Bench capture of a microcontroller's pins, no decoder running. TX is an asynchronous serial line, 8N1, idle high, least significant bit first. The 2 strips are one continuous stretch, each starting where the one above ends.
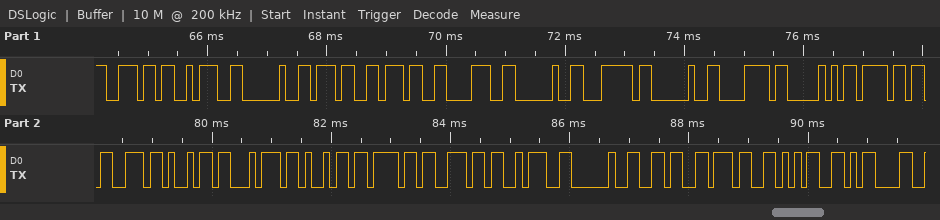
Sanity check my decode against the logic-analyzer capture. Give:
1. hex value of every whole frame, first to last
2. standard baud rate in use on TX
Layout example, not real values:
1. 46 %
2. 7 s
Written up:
1. 0x6E 0x3A 0x20 0x37 0x37 0x38 0x20 0x7C 0x20 0x78 0x50 0x6F 0x73 0x69 0x74 0x69 0x6F 0x6E 0x3A 0x20 0x36 0x37 0x35 0x0D
2. 9600 baud
